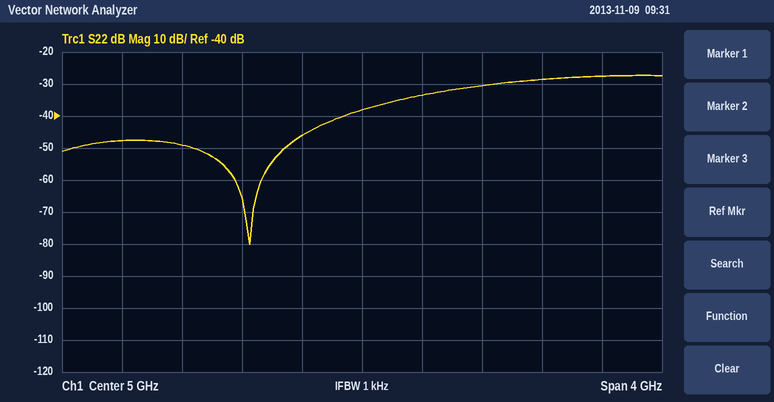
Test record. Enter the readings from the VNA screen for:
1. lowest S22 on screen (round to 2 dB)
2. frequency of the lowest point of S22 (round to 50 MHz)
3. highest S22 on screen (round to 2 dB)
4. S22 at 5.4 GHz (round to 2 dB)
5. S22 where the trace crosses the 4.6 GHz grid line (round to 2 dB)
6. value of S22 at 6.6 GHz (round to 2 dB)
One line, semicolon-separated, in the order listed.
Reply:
-80 dB; 4.25 GHz; -28 dB; -34 dB; -46 dB; -28 dB
